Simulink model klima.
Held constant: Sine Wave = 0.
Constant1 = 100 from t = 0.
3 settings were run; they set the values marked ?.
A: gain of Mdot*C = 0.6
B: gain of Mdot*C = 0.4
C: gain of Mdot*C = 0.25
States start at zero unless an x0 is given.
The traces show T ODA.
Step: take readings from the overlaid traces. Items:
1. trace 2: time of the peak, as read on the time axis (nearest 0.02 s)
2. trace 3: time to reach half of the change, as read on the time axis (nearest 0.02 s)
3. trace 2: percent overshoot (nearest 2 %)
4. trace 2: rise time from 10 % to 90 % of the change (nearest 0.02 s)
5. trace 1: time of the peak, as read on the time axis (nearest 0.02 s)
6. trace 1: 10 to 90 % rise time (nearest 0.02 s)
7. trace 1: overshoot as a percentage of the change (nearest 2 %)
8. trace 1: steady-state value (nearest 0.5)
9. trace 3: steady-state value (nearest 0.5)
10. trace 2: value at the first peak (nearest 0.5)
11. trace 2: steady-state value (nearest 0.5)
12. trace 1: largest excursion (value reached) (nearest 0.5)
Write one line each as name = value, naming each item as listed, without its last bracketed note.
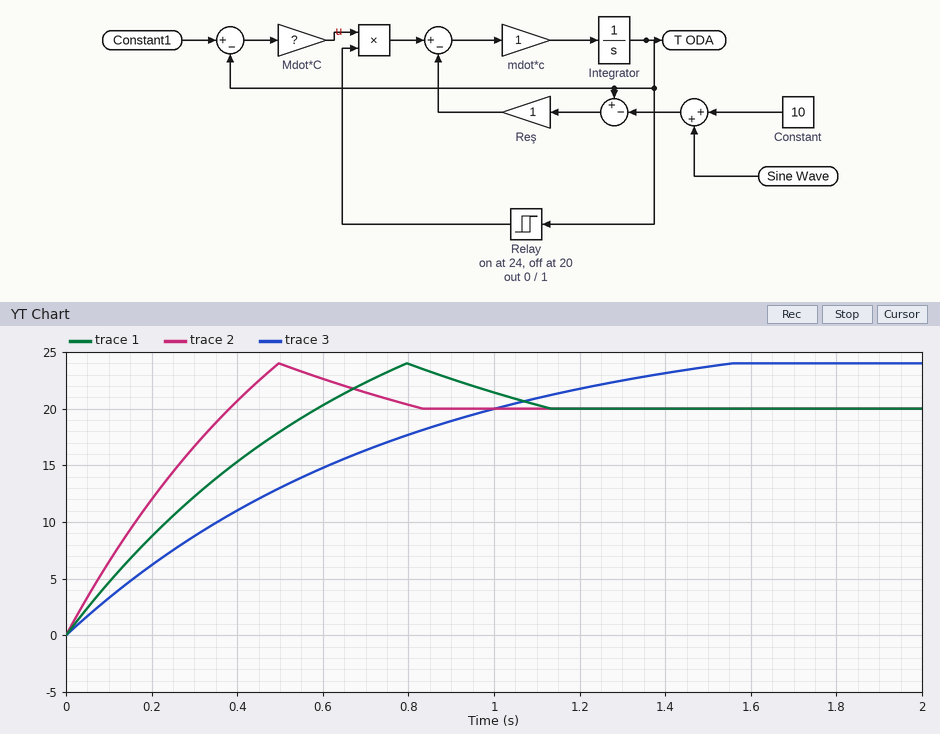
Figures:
trace 2: time of the peak, as read on the time axis = 0.50 s
trace 3: time to reach half of the change, as read on the time axis = 0.44 s
trace 2: percent overshoot = 20 %
trace 2: rise time from 10 % to 90 % of the change = 0.30 s
trace 1: time of the peak, as read on the time axis = 0.80 s
trace 1: 10 to 90 % rise time = 0.46 s
trace 1: overshoot as a percentage of the change = 20 %
trace 1: steady-state value = 20.0
trace 3: steady-state value = 24.0
trace 2: value at the first peak = 24.0
trace 2: steady-state value = 20.0
trace 1: largest excursion (value reached) = 24.0
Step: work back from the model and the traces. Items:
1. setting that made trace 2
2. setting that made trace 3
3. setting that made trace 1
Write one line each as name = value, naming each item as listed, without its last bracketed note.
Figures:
setting that made trace 2 = A
setting that made trace 3 = C
setting that made trace 1 = B
